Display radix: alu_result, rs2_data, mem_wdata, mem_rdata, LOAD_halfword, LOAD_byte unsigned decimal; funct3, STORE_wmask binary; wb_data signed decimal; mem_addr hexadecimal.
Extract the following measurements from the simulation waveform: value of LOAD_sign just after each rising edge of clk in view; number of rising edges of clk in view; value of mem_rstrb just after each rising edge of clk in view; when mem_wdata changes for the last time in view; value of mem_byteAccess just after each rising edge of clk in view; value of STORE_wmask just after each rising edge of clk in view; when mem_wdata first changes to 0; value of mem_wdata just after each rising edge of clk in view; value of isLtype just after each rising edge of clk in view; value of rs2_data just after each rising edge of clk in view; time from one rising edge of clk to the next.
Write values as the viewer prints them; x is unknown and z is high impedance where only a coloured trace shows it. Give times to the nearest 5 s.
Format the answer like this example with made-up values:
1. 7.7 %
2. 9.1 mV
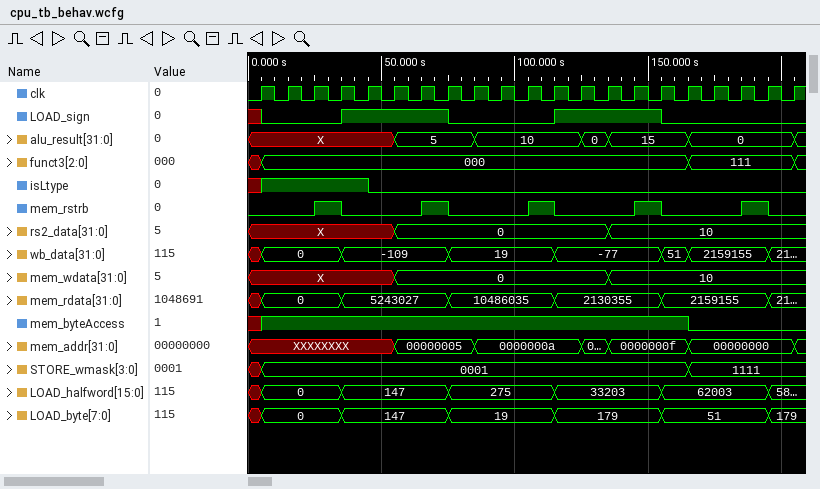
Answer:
1. 0 0 0 1 1 1 1 0 0 0 0 1 1 1 1 0 0 0 0 0 0
2. 21
3. 0 0 1 0 0 0 1 0 0 0 1 0 0 0 1 0 0 0 1 0 0
4. 135 s
5. 1 1 1 1 1 1 1 1 1 1 1 1 1 1 1 1 0 0 0 0 0
6. 0001, 0001, 0001, 0001, 0001, 0001, 0001, 0001, 0001, 0001, 0001, 0001, 0001, 0001, 0001, 0001, 1111, 1111, 1111, 1111, 1111
7. 55 s
8. X, X, X, X, X, 0, 0, 0, 0, 0, 0, 0, 0, 10, 10, 10, 10, 10, 10, 10, 10
9. 1 1 1 1 0 0 0 0 0 0 0 0 0 0 0 0 0 0 0 0 0
10. X, X, X, X, X, 0, 0, 0, 0, 0, 0, 0, 0, 10, 10, 10, 10, 10, 10, 10, 10
11. 10 s
